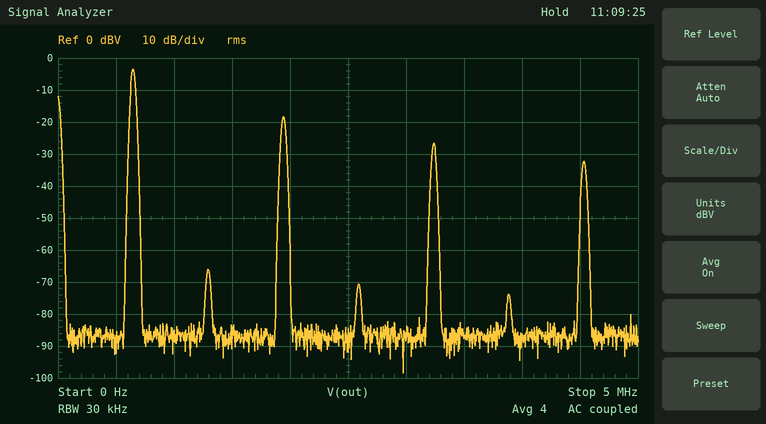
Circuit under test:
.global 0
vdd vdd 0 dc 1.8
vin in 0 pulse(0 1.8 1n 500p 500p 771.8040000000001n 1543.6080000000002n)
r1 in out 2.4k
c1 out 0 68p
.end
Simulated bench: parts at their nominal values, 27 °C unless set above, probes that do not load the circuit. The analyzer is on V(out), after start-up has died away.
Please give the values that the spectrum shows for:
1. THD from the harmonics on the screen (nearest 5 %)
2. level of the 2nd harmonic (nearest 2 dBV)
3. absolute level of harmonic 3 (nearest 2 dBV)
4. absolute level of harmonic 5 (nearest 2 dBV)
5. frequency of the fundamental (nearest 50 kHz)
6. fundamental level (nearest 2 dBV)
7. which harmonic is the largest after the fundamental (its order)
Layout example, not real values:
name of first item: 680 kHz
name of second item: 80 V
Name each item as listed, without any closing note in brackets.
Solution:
THD from the harmonics on the screen: 20 %
level of the 2nd harmonic: -66 dBV
absolute level of harmonic 3: -18 dBV
absolute level of harmonic 5: -26 dBV
frequency of the fundamental: 650 kHz
fundamental level: -4 dBV
which harmonic is the largest after the fundamental: 3
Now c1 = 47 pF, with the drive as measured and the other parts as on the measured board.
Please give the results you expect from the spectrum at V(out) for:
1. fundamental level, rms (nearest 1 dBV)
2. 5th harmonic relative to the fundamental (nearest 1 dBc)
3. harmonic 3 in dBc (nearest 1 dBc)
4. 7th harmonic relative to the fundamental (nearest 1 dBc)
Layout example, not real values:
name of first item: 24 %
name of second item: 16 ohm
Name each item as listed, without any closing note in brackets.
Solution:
fundamental level, rms: -3 dBV
5th harmonic relative to the fundamental: -21 dBc
harmonic 3 in dBc: -13 dBc
7th harmonic relative to the fundamental: -27 dBc
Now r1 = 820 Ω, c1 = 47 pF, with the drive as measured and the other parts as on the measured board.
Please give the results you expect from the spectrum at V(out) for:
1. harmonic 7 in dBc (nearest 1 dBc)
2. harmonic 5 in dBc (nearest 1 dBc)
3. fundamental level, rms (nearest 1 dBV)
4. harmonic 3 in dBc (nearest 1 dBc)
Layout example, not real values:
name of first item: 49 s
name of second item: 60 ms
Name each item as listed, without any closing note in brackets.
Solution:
harmonic 7 in dBc: -20 dBc
harmonic 5 in dBc: -16 dBc
fundamental level, rms: -2 dBV
harmonic 3 in dBc: -10 dBc
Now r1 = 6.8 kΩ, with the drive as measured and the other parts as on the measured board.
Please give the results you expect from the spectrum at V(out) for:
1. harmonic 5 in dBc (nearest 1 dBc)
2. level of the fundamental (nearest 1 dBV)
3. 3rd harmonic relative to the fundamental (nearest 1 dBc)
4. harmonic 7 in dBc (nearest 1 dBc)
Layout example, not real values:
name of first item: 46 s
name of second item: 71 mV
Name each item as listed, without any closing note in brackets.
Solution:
harmonic 5 in dBc: -27 dBc
level of the fundamental: -8 dBV
3rd harmonic relative to the fundamental: -18 dBc
harmonic 7 in dBc: -33 dBc
